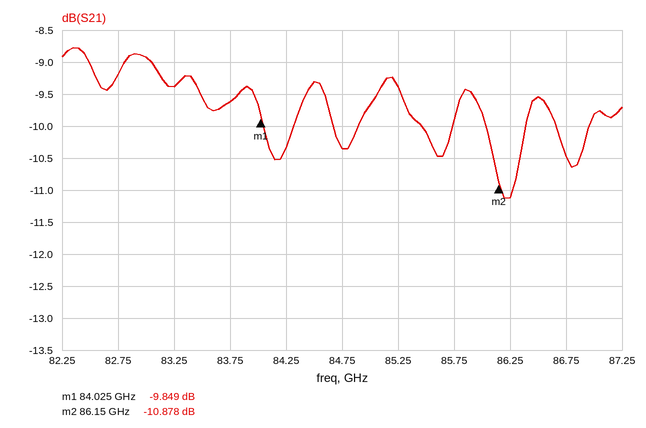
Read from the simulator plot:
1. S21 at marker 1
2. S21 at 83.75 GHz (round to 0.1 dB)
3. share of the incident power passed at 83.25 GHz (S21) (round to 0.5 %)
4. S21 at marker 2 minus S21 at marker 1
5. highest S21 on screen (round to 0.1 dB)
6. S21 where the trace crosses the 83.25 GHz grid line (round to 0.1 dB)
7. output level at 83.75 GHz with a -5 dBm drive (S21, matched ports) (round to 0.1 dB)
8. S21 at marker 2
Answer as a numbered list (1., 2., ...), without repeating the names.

1. -9.849 dB
2. -9.6 dB
3. 11.5 %
4. -1.029 dB
5. -8.8 dB
6. -9.4 dB
7. -14.6 dBm
8. -10.878 dB
